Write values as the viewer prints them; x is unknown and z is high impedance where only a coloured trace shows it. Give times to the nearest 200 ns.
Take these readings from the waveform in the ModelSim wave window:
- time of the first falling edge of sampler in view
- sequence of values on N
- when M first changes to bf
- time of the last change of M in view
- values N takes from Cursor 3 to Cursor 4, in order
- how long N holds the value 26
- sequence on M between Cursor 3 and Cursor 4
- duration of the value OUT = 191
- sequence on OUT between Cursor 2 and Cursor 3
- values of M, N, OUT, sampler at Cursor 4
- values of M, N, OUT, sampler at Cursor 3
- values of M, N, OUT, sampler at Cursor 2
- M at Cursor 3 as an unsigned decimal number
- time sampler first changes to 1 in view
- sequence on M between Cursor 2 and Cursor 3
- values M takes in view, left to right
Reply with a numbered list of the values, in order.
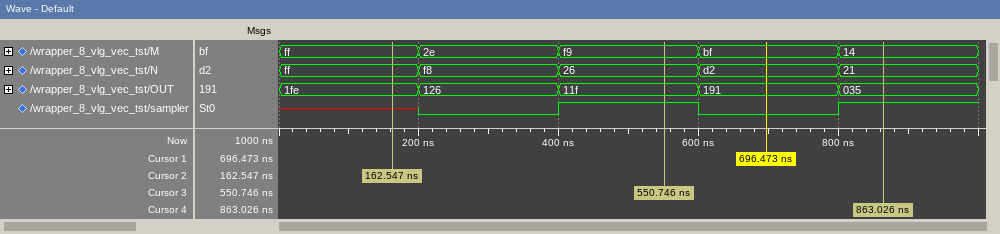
1. 600 ns
2. ff, f8, 26, d2, 21
3. 600 ns
4. 800 ns
5. 26, d2, 21
6. 200 ns
7. f9, bf, 14
8. 200 ns
9. 1fe, 126, 11f
10. M=14, N=21, OUT=035, sampler=1
11. M=f9, N=26, OUT=11f, sampler=1
12. M=ff, N=ff, OUT=1fe, sampler=x
13. 249
14. 400 ns
15. ff, 2e, f9
16. ff, 2e, f9, bf, 14
